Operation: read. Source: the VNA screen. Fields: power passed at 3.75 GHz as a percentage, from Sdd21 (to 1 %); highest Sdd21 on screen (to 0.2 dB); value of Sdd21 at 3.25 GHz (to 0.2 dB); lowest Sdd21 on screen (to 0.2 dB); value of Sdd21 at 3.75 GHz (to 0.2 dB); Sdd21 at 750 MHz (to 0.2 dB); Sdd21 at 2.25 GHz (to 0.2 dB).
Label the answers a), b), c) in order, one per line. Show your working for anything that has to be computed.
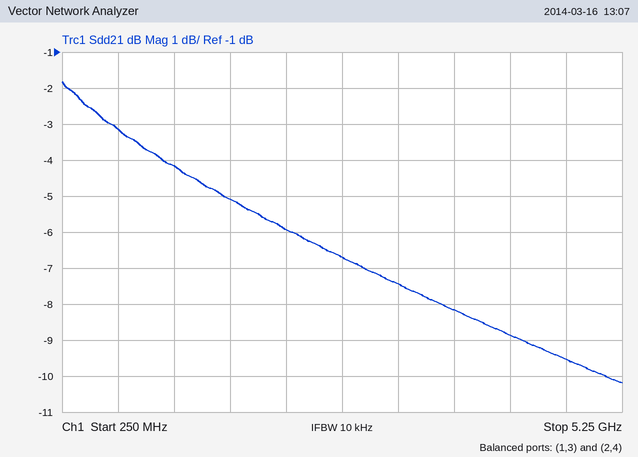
a) 10^(-8.2/10) ≈ 15 %
b) -1.8 dB
c) -7.4 dB
d) -10.2 dB
e) -8.2 dB
f) -3.2 dB
g) -6.0 dB
